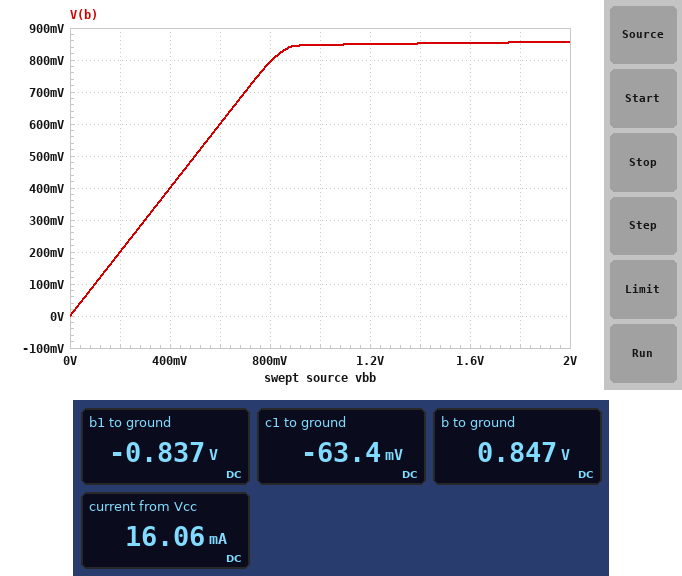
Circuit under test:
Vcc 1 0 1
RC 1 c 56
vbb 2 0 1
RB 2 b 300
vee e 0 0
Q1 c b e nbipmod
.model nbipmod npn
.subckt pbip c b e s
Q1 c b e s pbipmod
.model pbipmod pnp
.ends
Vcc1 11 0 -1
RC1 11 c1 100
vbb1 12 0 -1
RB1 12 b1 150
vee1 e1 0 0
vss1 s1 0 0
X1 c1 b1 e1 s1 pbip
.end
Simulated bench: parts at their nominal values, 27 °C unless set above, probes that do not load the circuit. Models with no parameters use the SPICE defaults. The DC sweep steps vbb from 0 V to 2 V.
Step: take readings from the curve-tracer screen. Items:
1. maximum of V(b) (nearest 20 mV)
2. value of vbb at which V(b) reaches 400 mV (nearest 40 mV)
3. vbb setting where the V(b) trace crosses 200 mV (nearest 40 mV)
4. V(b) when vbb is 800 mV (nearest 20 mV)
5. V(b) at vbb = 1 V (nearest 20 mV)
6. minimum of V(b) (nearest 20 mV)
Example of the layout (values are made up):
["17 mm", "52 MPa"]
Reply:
["860 mV", "400 mV", "200 mV", "800 mV", "840 mV", "0 V"]
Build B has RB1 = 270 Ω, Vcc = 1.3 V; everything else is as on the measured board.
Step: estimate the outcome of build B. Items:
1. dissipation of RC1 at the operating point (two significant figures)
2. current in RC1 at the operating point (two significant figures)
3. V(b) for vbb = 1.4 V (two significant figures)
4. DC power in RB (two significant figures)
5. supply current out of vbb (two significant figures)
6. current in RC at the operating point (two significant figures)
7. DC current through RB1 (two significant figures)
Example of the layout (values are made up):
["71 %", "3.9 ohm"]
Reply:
["8.5 mW", "9.2 mA", "860 mV", "71 µW", "490 µA", "21 mA", "610 µA"]
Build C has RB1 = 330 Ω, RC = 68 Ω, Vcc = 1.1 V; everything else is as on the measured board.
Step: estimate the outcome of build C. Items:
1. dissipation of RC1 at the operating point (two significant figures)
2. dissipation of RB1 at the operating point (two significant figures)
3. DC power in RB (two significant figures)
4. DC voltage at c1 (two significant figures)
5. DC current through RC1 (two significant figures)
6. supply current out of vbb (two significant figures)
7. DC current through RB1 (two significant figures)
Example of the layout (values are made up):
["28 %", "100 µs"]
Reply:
["8.4 mW", "84 µW", "80 µW", "-83 mV", "9.2 mA", "520 µA", "500 µA"]
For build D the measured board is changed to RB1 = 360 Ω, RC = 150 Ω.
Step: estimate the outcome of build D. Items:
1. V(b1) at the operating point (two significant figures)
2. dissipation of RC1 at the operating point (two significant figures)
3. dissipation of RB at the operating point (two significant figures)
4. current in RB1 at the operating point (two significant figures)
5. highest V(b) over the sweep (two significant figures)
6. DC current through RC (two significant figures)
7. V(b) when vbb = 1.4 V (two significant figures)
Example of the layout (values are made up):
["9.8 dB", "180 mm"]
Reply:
["-830 mV", "8.4 mW", "100 µW", "460 µA", "840 mV", "6.2 mA", "830 mV"]
